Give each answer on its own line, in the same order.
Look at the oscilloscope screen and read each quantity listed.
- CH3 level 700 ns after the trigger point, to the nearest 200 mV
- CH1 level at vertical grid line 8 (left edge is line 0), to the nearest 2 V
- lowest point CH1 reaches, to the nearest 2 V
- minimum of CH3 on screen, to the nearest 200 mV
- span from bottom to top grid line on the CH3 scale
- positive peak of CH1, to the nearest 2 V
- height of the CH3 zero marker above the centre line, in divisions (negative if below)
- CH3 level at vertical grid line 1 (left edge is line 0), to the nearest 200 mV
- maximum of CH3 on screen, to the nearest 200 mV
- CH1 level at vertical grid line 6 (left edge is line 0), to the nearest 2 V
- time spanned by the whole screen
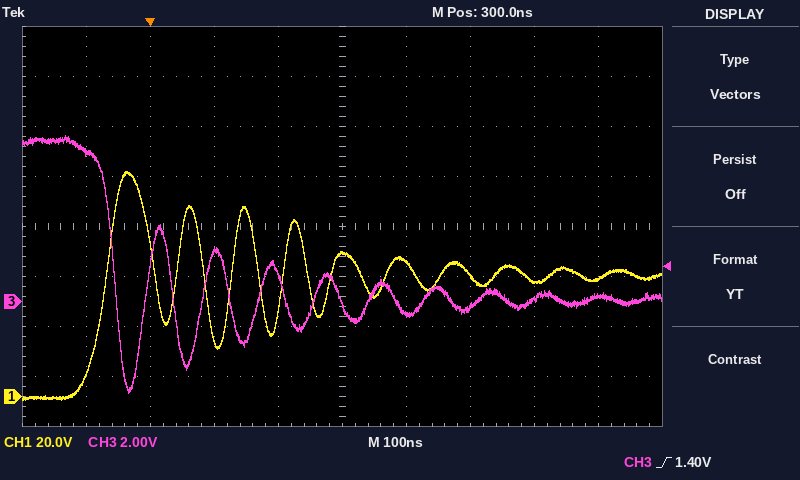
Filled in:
200 mV
46 V
-2 V
-3.6 V
16 V
90 V
-1.5 div
6.0 V
6.6 V
54 V
1 µs
